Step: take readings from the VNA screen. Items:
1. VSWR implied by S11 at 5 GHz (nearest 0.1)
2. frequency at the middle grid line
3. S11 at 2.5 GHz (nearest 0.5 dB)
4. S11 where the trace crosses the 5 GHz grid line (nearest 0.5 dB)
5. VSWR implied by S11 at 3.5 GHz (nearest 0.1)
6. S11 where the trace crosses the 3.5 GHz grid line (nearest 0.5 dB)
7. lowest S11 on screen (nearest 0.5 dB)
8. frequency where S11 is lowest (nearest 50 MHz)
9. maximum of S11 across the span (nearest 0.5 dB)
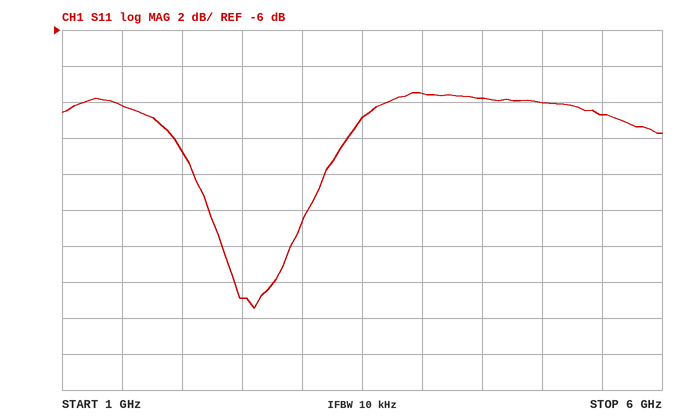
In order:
1.9
3.5 GHz
-21.0 dB
-10.0 dB
1.8
-11.0 dB
-21.5 dB
2.60 GHz
-9.5 dB
